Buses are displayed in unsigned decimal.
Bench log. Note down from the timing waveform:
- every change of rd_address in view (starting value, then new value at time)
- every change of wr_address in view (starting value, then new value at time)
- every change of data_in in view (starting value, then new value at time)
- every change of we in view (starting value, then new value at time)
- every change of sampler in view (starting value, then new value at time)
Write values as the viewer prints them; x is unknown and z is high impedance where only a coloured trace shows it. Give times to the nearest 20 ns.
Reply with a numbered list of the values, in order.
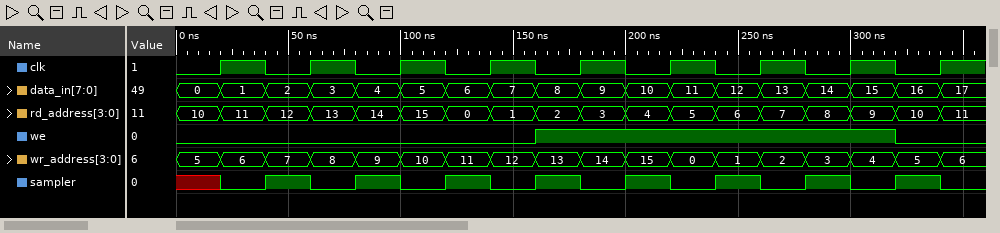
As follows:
1. 10, 11 at 20 ns, 12 at 40 ns, 13 at 60 ns, 14 at 80 ns, 15 at 100 ns, 0 at 120 ns, 1 at 140 ns, 2 at 160 ns, 3 at 180 ns, 4 at 200 ns, 5 at 220 ns, 6 at 240 ns, 7 at 260 ns, 8 at 280 ns, 9 at 300 ns, 10 at 320 ns, 11 at 340 ns
2. 5, 6 at 20 ns, 7 at 40 ns, 8 at 60 ns, 9 at 80 ns, 10 at 100 ns, 11 at 120 ns, 12 at 140 ns, 13 at 160 ns, 14 at 180 ns, 15 at 200 ns, 0 at 220 ns, 1 at 240 ns, 2 at 260 ns, 3 at 280 ns, 4 at 300 ns, 5 at 320 ns, 6 at 340 ns
3. 0, 1 at 20 ns, 2 at 40 ns, 3 at 60 ns, 4 at 80 ns, 5 at 100 ns, 6 at 120 ns, 7 at 140 ns, 8 at 160 ns, 9 at 180 ns, 10 at 200 ns, 11 at 220 ns, 12 at 240 ns, 13 at 260 ns, 14 at 280 ns, 15 at 300 ns, 16 at 320 ns, 17 at 340 ns
4. 0, 1 at 160 ns, 0 at 320 ns
5. x, 0 at 20 ns, 1 at 40 ns, 0 at 60 ns, 1 at 80 ns, 0 at 100 ns, 1 at 120 ns, 0 at 140 ns, 1 at 160 ns, 0 at 180 ns, 1 at 200 ns, 0 at 220 ns, 1 at 240 ns, 0 at 260 ns, 1 at 280 ns, 0 at 300 ns, 1 at 320 ns, 0 at 340 ns
